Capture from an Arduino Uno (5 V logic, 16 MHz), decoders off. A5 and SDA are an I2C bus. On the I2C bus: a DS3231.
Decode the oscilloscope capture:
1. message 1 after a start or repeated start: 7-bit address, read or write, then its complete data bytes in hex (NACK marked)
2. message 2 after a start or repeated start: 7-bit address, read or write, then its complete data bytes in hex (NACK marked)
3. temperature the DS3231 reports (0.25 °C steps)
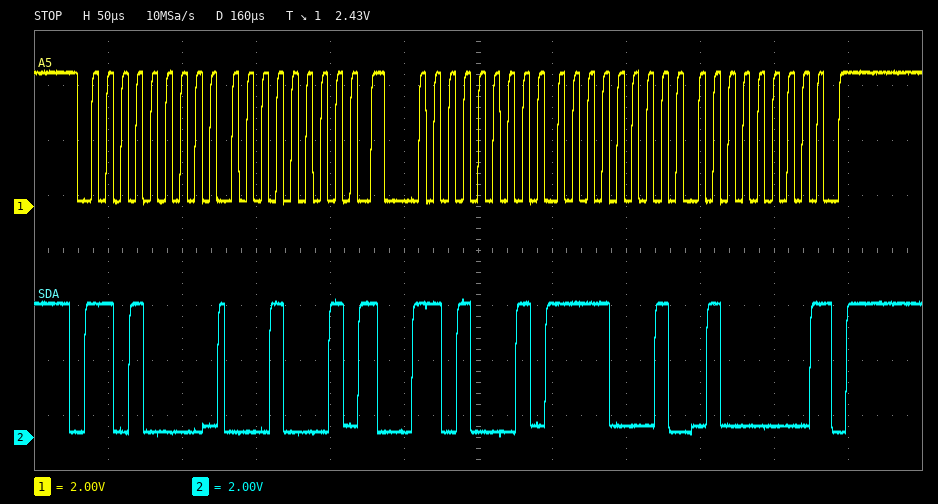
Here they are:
0x68 write: 11
0x68 read: F1 40 NACK
-14.75 °C
